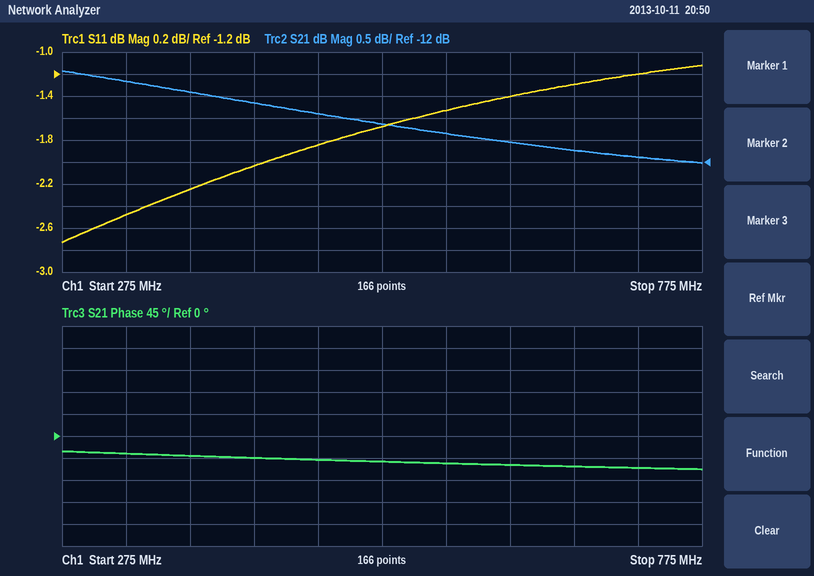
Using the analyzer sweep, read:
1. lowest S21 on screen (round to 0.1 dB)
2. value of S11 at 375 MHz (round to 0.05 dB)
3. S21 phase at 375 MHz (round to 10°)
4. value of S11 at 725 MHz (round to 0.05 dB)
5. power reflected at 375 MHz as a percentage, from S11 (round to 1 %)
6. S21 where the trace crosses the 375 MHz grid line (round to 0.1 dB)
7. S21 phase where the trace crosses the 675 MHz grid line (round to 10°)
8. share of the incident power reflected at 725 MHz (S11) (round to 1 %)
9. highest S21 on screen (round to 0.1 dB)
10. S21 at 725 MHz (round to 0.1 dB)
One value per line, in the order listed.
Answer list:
-12.0 dB
-2.25 dB
-40°
-1.20 dB
60 %
-10.4 dB
-60°
76 %
-9.9 dB
-11.9 dB
